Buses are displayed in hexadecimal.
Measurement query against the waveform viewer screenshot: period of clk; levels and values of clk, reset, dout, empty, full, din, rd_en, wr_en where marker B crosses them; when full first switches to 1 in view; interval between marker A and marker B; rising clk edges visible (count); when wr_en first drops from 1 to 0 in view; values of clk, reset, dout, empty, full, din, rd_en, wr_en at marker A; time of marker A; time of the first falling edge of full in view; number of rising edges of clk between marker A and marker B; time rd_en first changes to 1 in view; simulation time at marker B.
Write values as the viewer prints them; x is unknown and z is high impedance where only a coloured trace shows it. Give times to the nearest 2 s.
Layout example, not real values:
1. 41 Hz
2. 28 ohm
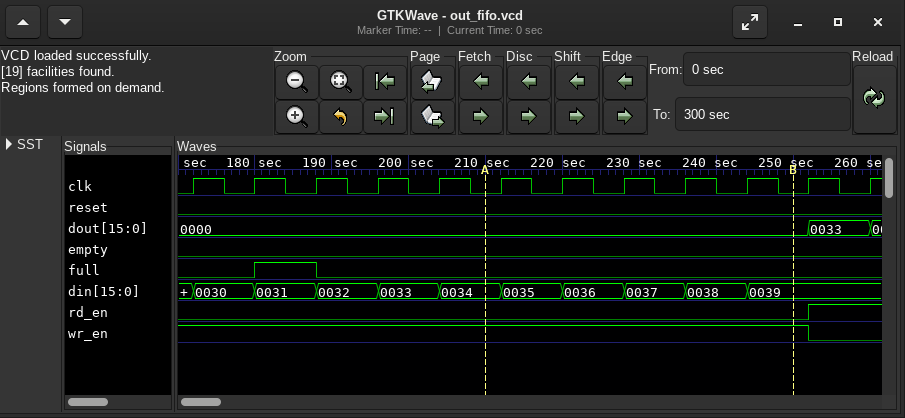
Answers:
1. 8 s
2. clk=0, reset=0, dout=0000, empty=0, full=0, din=0039, rd_en=0, wr_en=1
3. 180 s
4. 40 s
5. 12
6. 252 s
7. clk=0, reset=0, dout=0000, empty=0, full=0, din=0034, rd_en=0, wr_en=1
8. 210 s
9. 188 s
10. 5
11. 252 s
12. 250 s
